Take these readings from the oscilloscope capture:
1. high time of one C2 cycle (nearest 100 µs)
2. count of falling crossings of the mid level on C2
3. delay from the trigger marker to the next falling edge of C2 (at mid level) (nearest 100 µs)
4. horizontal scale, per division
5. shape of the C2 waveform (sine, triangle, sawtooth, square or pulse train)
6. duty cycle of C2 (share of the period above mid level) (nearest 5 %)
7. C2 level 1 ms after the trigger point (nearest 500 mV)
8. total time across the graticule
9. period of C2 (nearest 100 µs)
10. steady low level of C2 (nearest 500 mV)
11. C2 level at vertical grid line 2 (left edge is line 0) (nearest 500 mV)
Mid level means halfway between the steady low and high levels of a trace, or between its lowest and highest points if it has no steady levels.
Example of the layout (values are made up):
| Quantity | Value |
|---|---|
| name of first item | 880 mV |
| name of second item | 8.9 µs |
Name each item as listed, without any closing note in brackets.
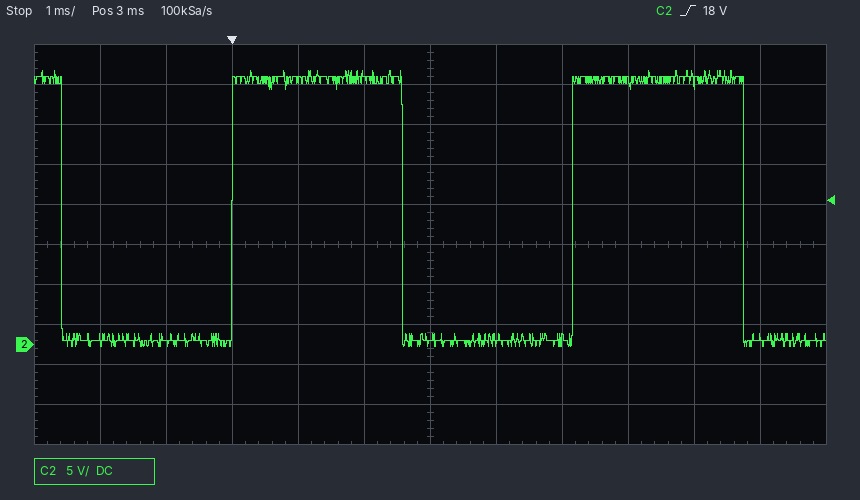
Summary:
| Quantity | Value |
|---|---|
| high time of one C2 cycle | 2.6 ms |
| count of falling crossings of the mid level on C2 | 3 |
| delay from the trigger marker to the next falling edge of C2 (at mid level) | 2.6 ms |
| horizontal scale, per division | 1 ms |
| shape of the C2 waveform | square |
| duty cycle of C2 (share of the period above mid level) | 50 % |
| C2 level 1 ms after the trigger point | 33.0 V |
| total time across the graticule | 12 ms |
| period of C2 | 5.2 ms |
| steady low level of C2 | 500 mV |
| C2 level at vertical grid line 2 (left edge is line 0) | 0.0 V |
